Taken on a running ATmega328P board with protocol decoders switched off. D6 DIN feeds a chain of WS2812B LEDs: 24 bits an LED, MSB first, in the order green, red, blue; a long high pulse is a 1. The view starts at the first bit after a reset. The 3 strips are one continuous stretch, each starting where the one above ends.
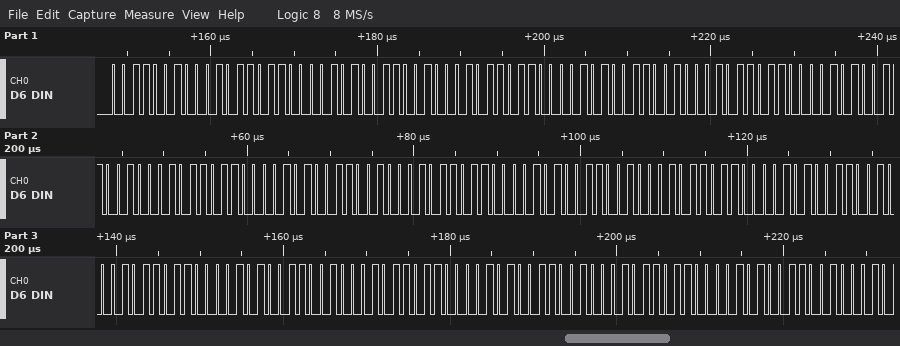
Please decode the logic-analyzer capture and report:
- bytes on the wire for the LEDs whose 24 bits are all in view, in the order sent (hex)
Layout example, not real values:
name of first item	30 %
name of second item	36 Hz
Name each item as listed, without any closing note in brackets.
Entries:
bytes on the wire for the LEDs whose 24 bits are all in view, in the order sent	32 2D 85 32 2D 85 32 2D 85 32 2D 85 32 2D 85 32 2D 85 32 2D 85 32 2D 85 32 2D 85
